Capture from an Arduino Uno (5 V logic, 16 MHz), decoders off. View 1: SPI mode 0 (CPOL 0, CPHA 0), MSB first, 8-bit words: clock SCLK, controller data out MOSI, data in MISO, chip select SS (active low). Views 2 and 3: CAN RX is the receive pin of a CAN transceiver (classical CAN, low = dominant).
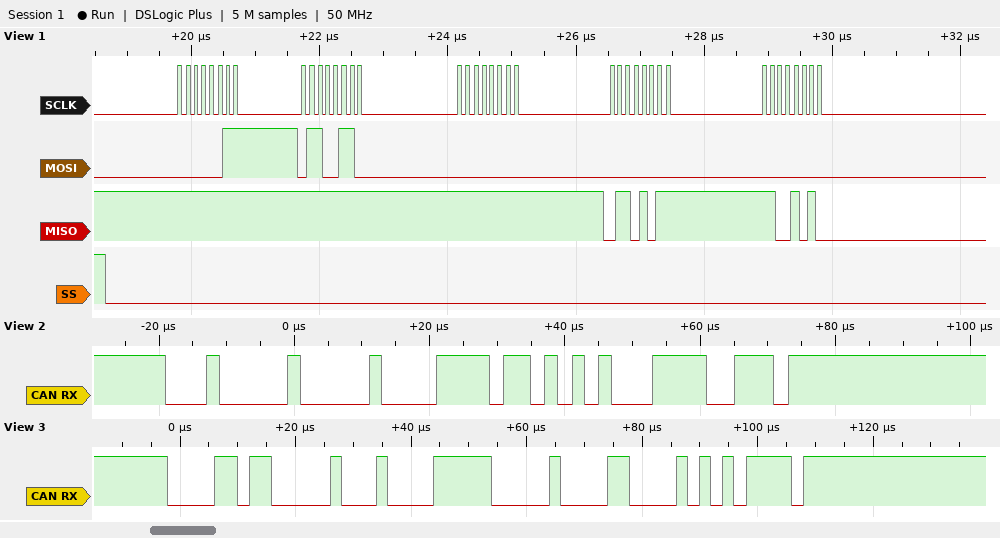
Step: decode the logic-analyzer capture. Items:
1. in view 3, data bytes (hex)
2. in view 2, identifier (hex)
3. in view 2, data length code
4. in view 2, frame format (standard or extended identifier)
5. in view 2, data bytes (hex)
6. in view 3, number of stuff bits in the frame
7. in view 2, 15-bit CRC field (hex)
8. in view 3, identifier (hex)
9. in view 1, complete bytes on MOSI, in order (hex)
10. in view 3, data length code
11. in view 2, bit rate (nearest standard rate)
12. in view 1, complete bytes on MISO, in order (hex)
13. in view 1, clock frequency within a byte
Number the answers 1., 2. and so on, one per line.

1. 1F 00
2. 0x100
3. 1
4. standard
5. ED
6. 3
7. 0x28F3
8. 0x0D8
9. 03 66 00 00 00
10. 2
11. 500 kbit/s
12. FF FF FF 6B CA
13. 8 MHz
